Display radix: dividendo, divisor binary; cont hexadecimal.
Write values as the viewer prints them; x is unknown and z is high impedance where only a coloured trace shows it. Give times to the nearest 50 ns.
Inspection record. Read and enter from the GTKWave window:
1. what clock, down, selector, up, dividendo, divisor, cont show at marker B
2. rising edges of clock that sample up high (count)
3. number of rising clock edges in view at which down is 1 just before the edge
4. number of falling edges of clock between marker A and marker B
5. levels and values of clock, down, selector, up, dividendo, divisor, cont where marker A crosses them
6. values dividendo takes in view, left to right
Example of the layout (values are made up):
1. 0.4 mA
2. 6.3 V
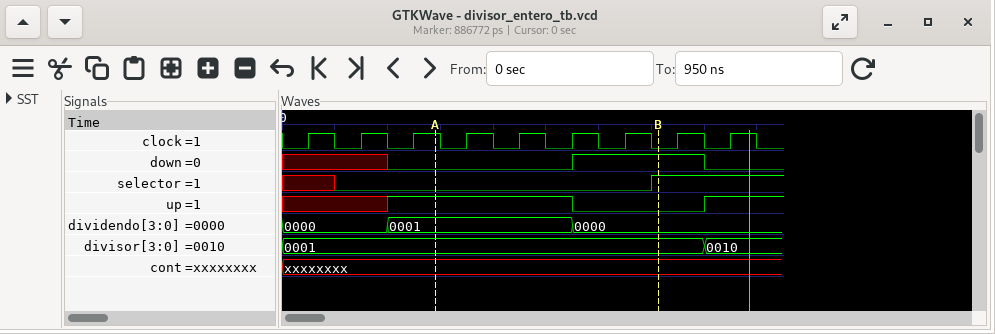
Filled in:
1. clock=0, down=1, selector=1, up=0, dividendo=0000, divisor=0001, cont=xxxxxxxx
2. 5
3. 2
4. 5
5. clock=1, down=0, selector=0, up=1, dividendo=0001, divisor=0001, cont=xxxxxxxx
6. 0000, 0001, 0000
